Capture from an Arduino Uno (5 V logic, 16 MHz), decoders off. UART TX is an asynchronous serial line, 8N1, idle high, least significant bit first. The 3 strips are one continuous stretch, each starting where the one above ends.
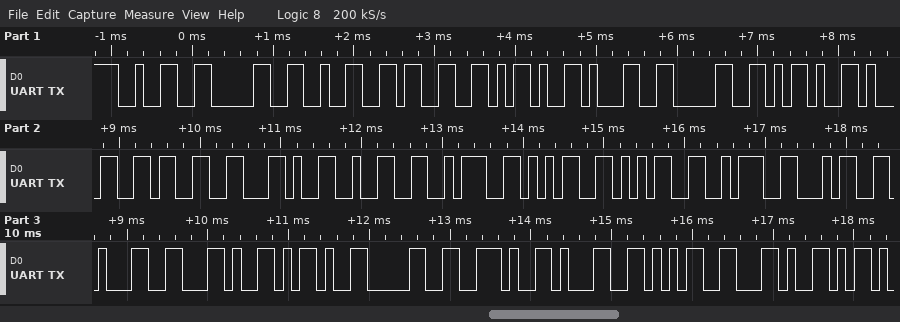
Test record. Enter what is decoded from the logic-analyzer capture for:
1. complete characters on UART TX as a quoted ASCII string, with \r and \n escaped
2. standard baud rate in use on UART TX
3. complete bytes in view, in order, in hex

"2023-10-13,2:55:41,-0.15,"
9600 baud
32 30 32 33 2D 31 30 2D 31 33 2C 32 3A 35 35 3A 34 31 2C 2D 30 2E 31 35 2C
